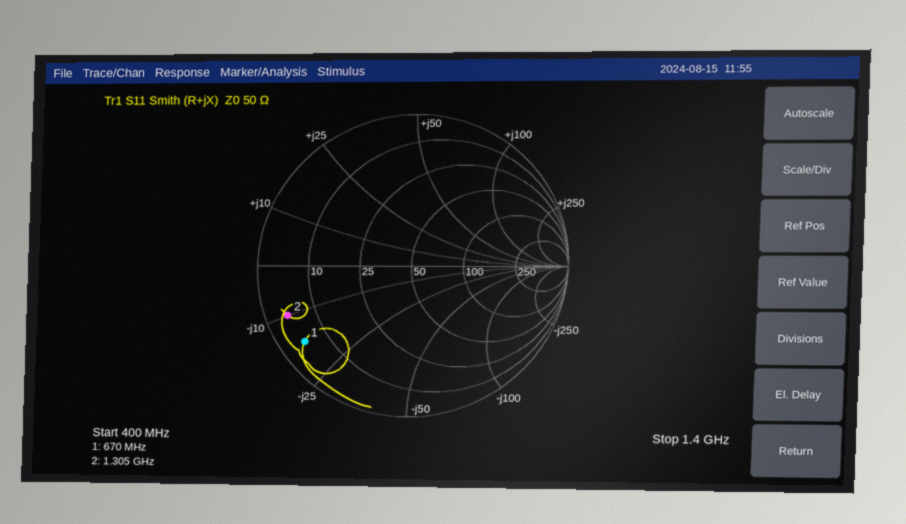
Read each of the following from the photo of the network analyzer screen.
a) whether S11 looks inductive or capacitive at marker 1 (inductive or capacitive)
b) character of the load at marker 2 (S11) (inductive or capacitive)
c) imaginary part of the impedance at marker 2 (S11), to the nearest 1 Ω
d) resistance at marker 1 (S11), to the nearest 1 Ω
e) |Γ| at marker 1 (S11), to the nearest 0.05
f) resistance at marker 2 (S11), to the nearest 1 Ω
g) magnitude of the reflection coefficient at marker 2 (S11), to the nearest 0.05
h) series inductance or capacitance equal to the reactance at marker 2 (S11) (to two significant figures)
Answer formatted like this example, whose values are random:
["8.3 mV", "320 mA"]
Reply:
["capacitive", "capacitive", "-10 Ω", "5 Ω", "0.85", "4 Ω", "0.85", "12 pF"]
